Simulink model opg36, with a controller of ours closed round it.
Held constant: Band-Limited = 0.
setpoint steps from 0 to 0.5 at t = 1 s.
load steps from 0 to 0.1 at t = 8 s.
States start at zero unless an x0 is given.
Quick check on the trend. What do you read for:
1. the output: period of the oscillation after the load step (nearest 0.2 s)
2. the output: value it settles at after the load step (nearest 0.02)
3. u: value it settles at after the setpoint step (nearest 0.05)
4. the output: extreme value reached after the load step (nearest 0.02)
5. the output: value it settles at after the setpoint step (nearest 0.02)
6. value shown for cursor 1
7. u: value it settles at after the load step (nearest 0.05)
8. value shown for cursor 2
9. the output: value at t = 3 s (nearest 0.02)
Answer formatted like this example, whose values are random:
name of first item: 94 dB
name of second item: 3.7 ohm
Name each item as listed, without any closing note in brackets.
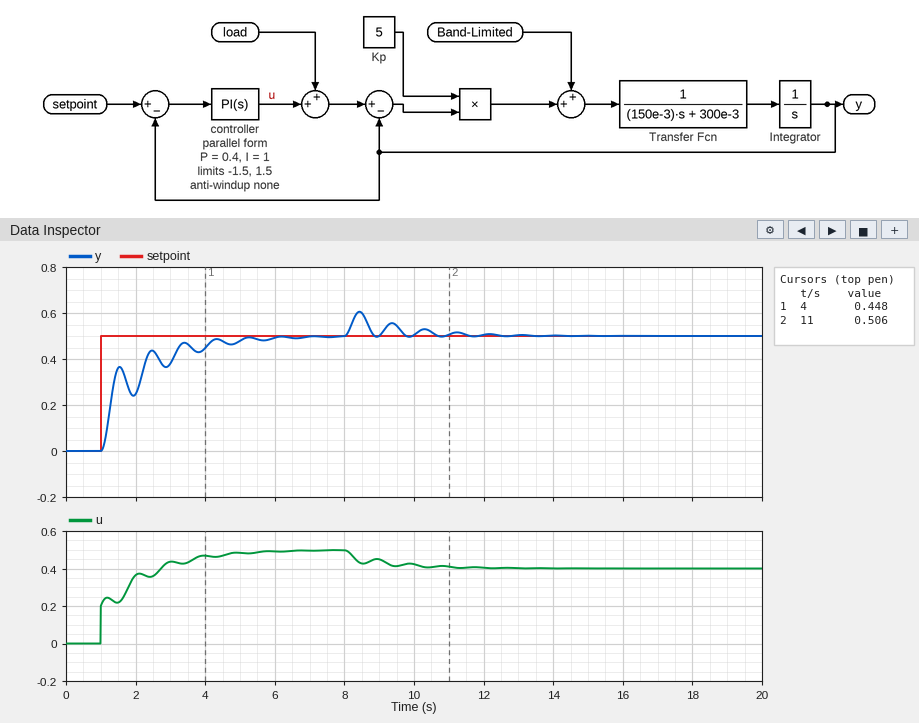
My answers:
the output: period of the oscillation after the load step: 1.0 s
the output: value it settles at after the load step: 0.50
u: value it settles at after the setpoint step: 0.50
the output: extreme value reached after the load step: 0.60
the output: value it settles at after the setpoint step: 0.50
value shown for cursor 1: 0.448
u: value it settles at after the load step: 0.40
value shown for cursor 2: 0.506
the output: value at t = 3 s: 0.38
